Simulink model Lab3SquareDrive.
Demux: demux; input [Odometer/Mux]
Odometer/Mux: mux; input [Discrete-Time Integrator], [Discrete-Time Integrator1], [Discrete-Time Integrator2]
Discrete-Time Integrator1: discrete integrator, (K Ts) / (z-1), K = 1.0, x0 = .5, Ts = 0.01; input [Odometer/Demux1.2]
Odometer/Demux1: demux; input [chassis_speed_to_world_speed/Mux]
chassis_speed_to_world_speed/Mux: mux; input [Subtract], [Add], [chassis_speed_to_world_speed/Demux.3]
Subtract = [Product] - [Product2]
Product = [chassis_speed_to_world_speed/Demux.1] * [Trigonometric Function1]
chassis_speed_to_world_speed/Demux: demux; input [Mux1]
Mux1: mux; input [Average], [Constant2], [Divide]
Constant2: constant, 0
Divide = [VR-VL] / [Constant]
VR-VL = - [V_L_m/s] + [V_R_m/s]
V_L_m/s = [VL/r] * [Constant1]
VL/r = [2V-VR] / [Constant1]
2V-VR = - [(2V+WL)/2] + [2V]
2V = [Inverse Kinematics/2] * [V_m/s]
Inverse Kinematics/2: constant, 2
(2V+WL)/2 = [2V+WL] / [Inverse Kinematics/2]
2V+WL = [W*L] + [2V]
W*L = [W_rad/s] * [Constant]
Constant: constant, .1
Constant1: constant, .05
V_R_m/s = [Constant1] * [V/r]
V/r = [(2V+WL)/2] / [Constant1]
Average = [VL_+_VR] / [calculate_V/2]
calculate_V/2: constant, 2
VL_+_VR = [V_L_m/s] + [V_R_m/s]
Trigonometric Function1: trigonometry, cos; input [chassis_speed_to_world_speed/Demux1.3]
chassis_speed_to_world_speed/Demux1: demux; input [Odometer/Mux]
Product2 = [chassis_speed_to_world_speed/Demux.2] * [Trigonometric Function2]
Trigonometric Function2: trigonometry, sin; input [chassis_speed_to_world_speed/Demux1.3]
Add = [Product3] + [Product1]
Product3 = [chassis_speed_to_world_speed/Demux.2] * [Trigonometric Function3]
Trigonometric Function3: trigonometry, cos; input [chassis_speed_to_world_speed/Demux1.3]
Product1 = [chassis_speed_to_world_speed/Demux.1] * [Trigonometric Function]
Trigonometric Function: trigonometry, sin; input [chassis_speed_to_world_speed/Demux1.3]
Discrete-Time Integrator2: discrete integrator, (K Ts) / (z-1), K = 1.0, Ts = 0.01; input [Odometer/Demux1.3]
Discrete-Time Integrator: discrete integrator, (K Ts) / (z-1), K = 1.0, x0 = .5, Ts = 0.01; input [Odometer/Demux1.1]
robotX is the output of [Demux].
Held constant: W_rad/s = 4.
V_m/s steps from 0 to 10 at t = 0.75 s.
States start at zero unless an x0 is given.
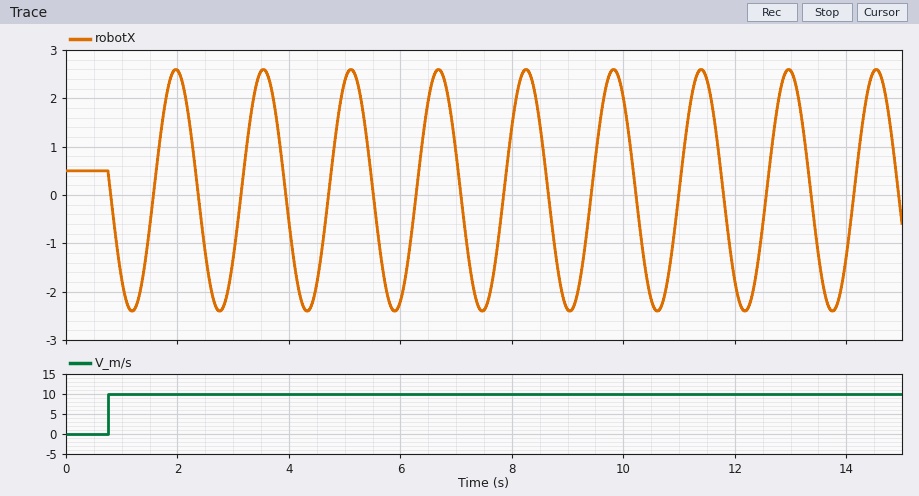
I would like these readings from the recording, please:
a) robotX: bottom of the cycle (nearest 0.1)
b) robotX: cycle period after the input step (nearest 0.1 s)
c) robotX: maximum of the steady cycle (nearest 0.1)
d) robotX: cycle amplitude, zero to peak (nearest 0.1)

-2.4
1.6 s
2.6
2.5
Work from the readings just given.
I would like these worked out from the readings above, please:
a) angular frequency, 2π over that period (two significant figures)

3.9 rad/s
